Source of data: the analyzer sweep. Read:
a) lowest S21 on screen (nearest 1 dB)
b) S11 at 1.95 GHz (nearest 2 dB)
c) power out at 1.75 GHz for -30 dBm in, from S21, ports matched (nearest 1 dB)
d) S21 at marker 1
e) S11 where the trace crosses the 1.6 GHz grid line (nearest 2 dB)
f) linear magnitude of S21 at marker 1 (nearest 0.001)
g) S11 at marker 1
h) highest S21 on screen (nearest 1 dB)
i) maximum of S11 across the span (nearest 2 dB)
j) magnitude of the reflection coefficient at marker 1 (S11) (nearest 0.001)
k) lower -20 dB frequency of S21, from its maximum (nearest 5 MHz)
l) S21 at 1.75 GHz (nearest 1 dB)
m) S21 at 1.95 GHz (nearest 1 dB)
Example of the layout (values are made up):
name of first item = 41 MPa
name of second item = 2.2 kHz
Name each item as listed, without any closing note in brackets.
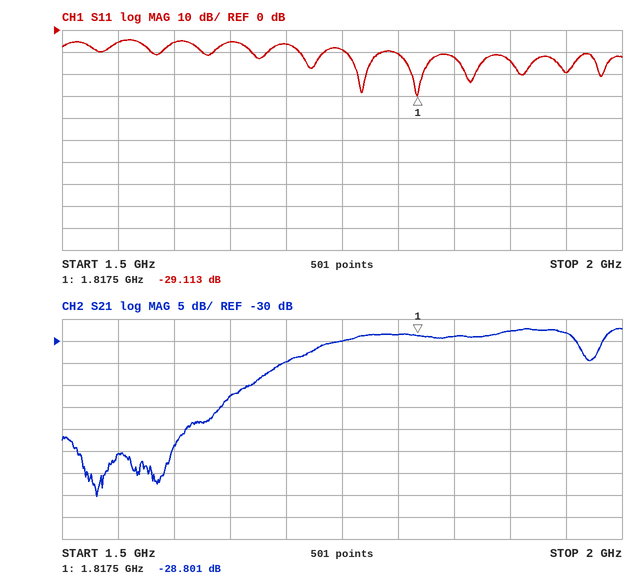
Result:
lowest S21 on screen = -65 dB
S11 at 1.95 GHz = -20 dB
power out at 1.75 GHz for -30 dBm in, from S21, ports matched = -60 dBm
S21 at marker 1 = -28.801 dB
S11 where the trace crosses the 1.6 GHz grid line = -6 dB
linear magnitude of S21 at marker 1 = 0.036
S11 at marker 1 = -29.113 dB
highest S21 on screen = -27 dB
maximum of S11 across the span = -4 dB
magnitude of the reflection coefficient at marker 1 (S11) = 0.035
lower -20 dB frequency of S21, from its maximum = 1.635 GHz
S21 at 1.75 GHz = -30 dB
S21 at 1.95 GHz = -28 dB
